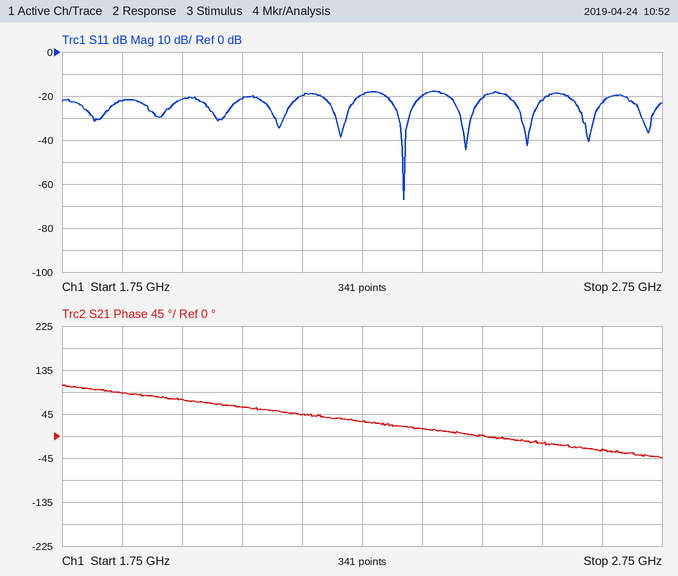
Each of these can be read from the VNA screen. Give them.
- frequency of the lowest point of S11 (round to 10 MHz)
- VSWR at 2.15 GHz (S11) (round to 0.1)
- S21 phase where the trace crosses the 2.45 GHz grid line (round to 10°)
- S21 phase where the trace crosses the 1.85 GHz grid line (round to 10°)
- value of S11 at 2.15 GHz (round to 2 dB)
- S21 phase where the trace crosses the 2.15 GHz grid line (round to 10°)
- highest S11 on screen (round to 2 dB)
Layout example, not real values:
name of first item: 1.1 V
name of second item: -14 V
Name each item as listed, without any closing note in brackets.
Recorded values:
frequency of the lowest point of S11: 2.32 GHz
VSWR at 2.15 GHz (S11): 1.2
S21 phase where the trace crosses the 2.45 GHz grid line: 0°
S21 phase where the trace crosses the 1.85 GHz grid line: 90°
value of S11 at 2.15 GHz: -20 dB
S21 phase where the trace crosses the 2.15 GHz grid line: 40°
highest S11 on screen: -18 dB
